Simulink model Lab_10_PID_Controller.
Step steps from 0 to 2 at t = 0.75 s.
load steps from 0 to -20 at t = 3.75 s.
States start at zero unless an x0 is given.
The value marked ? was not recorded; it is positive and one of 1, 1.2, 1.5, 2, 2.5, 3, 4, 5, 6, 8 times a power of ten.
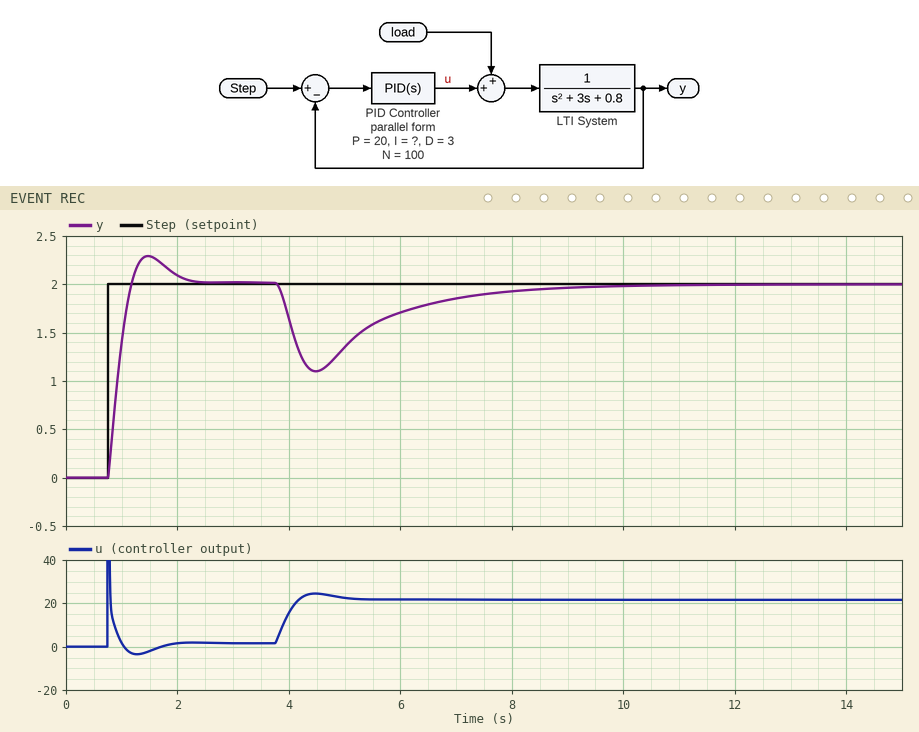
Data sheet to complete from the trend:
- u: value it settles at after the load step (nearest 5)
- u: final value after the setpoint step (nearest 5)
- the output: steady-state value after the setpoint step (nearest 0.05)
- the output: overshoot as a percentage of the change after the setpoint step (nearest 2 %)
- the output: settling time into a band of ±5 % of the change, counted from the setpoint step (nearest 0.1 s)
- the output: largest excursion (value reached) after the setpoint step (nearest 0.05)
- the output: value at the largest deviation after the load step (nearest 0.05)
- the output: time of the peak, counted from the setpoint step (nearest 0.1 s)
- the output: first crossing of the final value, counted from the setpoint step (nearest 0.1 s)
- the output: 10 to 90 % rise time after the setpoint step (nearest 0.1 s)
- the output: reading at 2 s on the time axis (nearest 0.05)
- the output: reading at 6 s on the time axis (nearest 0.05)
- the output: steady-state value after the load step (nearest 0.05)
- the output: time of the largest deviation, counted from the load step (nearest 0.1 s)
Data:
20
0
2.00
14 %
1.2 s
2.30
1.10
0.7 s
0.4 s
0.3 s
2.10
1.70
2.00
0.7 s
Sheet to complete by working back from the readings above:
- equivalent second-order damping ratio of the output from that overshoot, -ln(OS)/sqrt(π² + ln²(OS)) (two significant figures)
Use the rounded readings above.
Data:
0.53
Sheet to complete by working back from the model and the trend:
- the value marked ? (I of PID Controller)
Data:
12
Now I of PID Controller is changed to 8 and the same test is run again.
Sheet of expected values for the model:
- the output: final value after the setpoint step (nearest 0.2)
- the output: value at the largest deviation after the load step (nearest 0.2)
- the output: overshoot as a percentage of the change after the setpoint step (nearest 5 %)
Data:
2.0
1.0
10 %
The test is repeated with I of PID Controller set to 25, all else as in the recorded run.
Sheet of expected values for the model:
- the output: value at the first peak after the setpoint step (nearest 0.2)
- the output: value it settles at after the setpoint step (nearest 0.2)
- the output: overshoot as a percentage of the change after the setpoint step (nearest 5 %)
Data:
2.4
2.0
25 %
